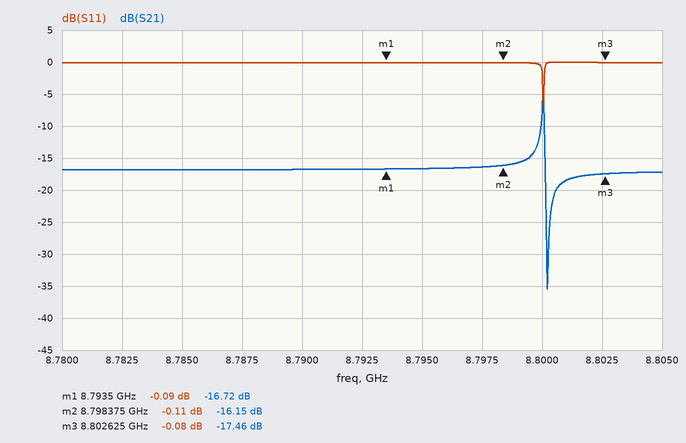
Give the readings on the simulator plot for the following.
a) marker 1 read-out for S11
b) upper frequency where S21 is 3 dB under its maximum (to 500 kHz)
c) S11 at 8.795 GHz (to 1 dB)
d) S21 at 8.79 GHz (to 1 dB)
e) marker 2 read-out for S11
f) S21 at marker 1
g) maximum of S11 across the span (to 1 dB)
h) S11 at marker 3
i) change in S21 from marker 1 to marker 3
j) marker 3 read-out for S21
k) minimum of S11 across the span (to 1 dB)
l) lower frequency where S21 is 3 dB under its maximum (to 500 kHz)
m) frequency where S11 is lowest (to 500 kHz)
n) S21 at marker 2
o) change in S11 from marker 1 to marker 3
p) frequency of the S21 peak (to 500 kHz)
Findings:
-0.09 dB
8.8000 GHz
0 dB
-17 dB
-0.11 dB
-16.72 dB
0 dB
-0.08 dB
-0.74 dB
-17.46 dB
-7 dB
8.8000 GHz
8.8000 GHz
-16.15 dB
0.01 dB
8.8000 GHz
